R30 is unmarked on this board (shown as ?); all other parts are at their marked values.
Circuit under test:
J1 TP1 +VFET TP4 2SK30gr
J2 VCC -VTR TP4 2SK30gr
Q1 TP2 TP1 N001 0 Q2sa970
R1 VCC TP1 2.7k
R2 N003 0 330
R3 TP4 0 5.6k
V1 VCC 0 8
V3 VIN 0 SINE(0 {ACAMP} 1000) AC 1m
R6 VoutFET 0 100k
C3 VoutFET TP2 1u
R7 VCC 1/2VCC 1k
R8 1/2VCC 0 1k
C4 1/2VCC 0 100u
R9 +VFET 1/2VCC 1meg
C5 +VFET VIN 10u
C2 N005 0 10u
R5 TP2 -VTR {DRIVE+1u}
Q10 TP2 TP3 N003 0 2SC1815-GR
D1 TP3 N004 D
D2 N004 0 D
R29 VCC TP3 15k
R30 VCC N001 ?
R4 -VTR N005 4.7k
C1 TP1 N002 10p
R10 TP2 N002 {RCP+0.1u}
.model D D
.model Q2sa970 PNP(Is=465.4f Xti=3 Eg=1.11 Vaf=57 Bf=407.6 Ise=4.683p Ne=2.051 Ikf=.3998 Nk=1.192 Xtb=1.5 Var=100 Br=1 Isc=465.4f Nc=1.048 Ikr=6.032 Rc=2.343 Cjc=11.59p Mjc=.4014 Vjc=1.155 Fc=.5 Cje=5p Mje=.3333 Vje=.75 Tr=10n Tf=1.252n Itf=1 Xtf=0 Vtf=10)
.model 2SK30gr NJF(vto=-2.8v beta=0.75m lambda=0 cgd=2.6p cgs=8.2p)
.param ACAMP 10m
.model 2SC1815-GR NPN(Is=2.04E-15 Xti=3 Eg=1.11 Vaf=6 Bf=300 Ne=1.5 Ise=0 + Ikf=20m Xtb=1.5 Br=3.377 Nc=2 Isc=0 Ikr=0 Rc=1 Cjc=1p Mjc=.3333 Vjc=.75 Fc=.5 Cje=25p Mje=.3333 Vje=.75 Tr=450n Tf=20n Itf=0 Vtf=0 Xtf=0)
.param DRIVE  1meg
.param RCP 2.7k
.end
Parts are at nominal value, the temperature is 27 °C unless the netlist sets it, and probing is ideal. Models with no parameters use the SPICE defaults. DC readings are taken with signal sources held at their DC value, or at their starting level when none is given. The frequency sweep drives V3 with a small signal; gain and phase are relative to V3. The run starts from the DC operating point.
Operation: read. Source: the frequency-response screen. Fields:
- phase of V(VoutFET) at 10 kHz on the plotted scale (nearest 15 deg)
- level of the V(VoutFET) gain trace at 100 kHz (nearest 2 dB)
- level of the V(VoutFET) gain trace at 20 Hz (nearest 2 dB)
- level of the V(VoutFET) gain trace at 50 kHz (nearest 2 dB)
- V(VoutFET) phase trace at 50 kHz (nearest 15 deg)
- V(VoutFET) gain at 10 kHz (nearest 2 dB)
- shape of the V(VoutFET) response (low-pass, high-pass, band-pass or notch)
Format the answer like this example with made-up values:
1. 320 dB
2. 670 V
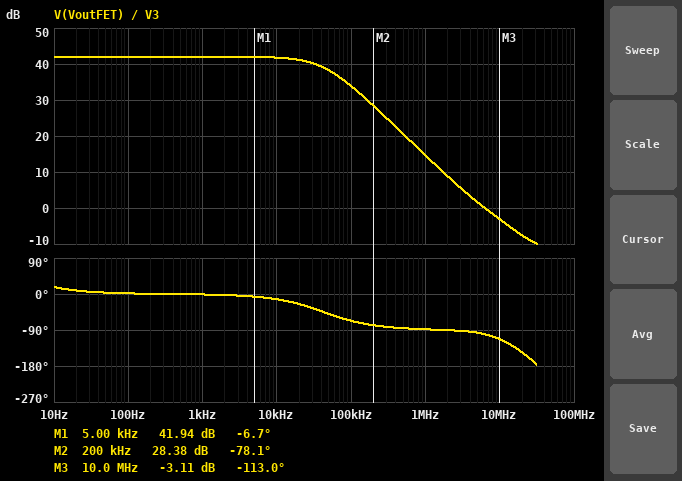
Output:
1. -15 deg
2. 34 dB
3. 42 dB
4. 38 dB
5. -45 deg
6. 42 dB
7. low-pass
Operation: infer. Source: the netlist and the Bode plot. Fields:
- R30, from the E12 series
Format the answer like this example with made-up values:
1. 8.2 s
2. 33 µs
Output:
1. 270 Ω
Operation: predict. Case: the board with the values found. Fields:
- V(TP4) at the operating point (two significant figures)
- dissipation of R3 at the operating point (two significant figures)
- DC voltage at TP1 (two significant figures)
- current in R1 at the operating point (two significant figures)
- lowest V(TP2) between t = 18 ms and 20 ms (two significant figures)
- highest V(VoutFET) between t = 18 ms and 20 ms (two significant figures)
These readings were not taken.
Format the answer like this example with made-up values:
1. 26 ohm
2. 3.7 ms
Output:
1. 6.1 V
2. 6.6 mW
3. 7.0 V
4. 380 µA
5. 3.0 V
6. 1.3 V
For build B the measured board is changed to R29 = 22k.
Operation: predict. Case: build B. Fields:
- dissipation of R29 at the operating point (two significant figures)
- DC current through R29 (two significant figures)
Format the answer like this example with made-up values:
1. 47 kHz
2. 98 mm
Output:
1. 2.1 mW
2. 310 µA
